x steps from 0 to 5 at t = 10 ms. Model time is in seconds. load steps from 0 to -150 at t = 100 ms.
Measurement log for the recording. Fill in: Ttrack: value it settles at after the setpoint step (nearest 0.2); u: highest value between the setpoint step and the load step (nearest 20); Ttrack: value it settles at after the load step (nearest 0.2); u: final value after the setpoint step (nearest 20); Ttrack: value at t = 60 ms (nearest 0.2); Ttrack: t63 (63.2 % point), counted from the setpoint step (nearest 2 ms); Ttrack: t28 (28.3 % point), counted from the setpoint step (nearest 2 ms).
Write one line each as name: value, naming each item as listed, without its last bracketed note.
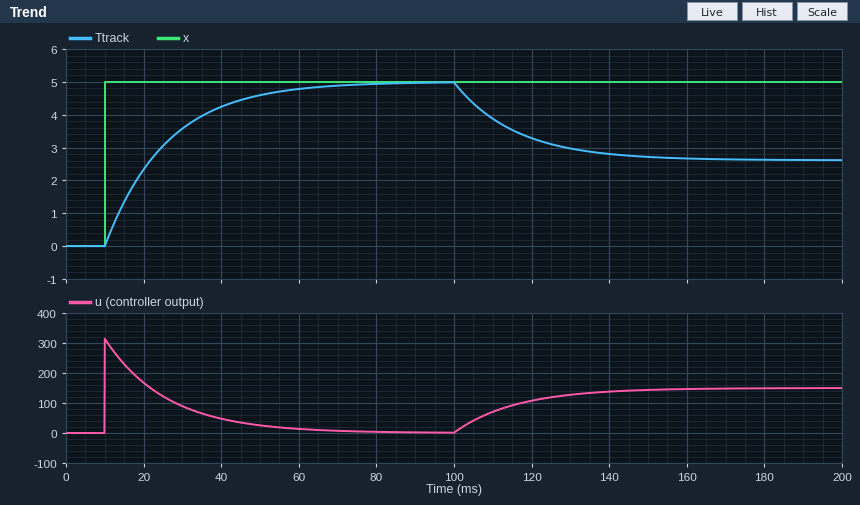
Ttrack: value it settles at after the setpoint step: 5.0
u: highest value between the setpoint step and the load step: 320
Ttrack: value it settles at after the load step: 2.6
u: final value after the setpoint step: 0
Ttrack: value at t = 60 ms: 4.8
Ttrack: t63 (63.2 % point), counted from the setpoint step: 16 ms
Ttrack: t28 (28.3 % point), counted from the setpoint step: 6 ms
